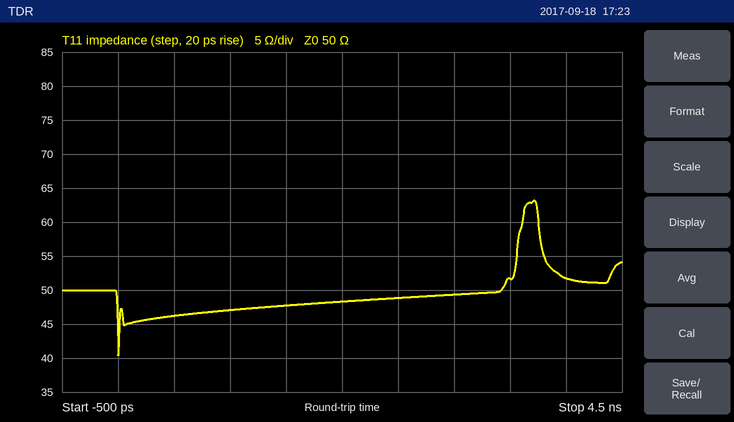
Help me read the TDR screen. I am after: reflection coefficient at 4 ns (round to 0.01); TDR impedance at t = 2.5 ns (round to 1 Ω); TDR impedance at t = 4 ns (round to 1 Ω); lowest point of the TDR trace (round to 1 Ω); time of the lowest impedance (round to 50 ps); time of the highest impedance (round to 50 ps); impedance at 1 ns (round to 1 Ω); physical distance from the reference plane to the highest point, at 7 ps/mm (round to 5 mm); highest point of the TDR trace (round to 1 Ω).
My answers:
+0.02
49 Ω
52 Ω
40 Ω
0 ps
3.70 ns
47 Ω
265 mm
63 Ω
